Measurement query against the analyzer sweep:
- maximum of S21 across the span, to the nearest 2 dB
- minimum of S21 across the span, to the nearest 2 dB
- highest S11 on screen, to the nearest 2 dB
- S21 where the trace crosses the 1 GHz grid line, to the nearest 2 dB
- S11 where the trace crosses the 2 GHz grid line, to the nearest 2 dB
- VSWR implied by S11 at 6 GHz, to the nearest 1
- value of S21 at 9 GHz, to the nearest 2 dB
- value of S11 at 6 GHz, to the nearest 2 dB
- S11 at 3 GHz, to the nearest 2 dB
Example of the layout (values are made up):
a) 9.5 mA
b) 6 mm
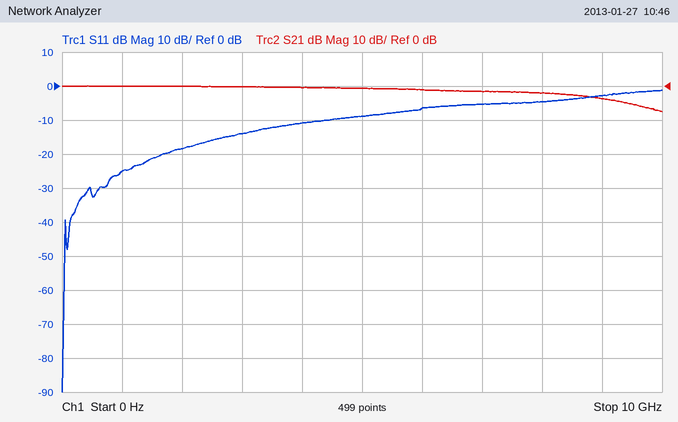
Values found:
a) 0 dB
b) -8 dB
c) -2 dB
d) 0 dB
e) -18 dB
f) 3
g) -4 dB
h) -6 dB
i) -14 dB
